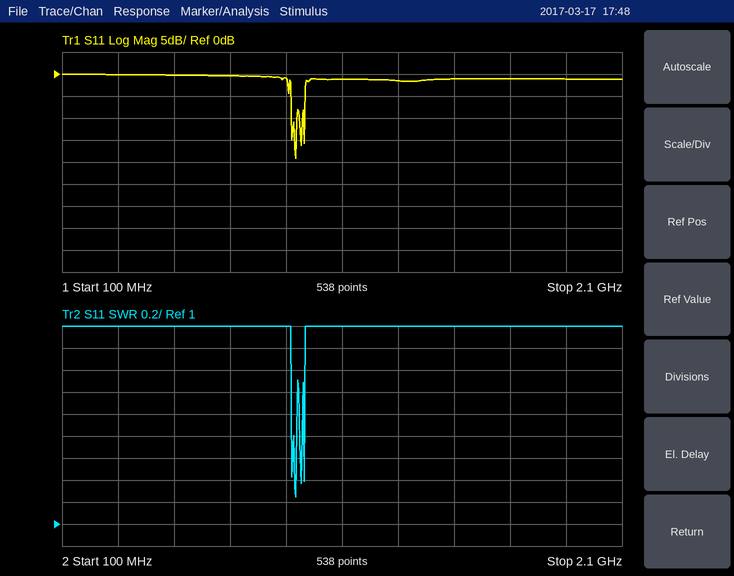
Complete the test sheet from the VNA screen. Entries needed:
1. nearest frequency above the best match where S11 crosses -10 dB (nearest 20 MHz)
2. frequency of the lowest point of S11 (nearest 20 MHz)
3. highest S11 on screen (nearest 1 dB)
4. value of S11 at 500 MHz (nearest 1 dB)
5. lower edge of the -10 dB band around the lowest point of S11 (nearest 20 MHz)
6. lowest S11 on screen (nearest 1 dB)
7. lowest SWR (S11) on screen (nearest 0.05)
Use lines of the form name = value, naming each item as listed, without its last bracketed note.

nearest frequency above the best match where S11 crosses -10 dB = 940 MHz
frequency of the lowest point of S11 = 940 MHz
highest S11 on screen = 0 dB
value of S11 at 500 MHz = 0 dB
lower edge of the -10 dB band around the lowest point of S11 = 920 MHz
lowest S11 on screen = -19 dB
lowest SWR (S11) on screen = 1.25
